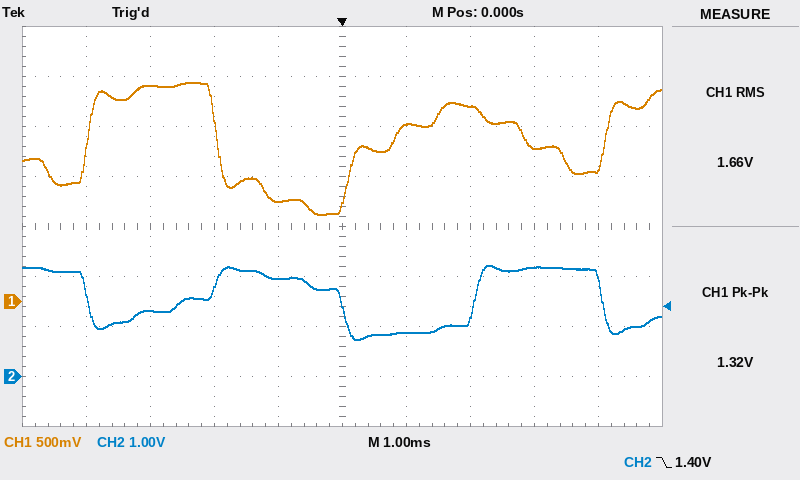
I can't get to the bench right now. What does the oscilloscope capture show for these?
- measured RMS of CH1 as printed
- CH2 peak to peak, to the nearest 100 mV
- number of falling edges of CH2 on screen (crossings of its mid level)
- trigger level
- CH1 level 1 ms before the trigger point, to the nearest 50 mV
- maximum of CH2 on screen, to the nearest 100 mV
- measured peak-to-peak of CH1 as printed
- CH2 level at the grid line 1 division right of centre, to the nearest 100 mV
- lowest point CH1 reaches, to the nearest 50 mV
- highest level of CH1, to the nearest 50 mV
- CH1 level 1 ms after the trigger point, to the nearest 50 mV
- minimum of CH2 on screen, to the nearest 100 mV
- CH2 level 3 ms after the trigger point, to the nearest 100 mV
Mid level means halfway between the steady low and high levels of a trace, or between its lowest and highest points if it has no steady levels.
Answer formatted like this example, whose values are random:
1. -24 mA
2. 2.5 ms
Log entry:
1. 1.66 V
2. 1.5 V
3. 3
4. 1.40 V
5. 1.00 V
6. 2.2 V
7. 1.32 V
8. 900 mV
9. 850 mV
10. 2.20 V
11. 1.75 V
12. 700 mV
13. 2.2 V
